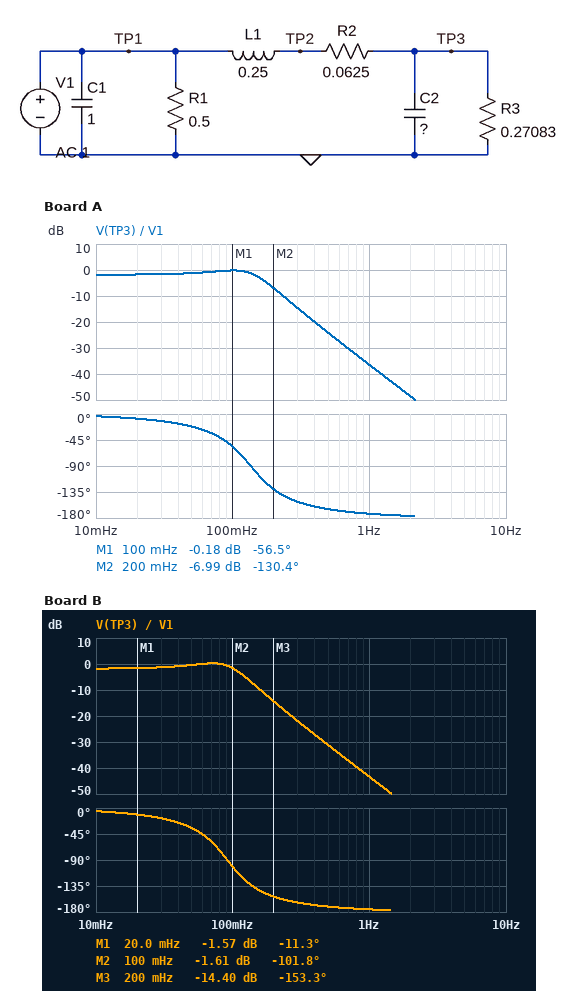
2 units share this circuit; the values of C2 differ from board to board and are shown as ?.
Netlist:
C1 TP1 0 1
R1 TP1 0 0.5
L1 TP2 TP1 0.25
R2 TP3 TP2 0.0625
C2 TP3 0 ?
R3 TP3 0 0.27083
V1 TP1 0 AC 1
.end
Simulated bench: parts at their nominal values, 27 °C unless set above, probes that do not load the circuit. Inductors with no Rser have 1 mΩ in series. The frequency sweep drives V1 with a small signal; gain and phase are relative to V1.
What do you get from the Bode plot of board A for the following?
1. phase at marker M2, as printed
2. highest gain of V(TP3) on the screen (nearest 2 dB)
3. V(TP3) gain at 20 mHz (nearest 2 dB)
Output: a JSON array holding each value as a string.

["-130.4 deg", "0 dB", "-2 dB"]
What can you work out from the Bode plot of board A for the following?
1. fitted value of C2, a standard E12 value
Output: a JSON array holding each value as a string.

["6.8 F"]
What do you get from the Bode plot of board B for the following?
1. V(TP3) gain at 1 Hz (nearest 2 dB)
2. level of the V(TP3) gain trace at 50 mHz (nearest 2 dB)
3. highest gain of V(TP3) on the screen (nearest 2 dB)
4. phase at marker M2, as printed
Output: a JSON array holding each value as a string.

["-44 dB", "0 dB", "0 dB", "-101.8 deg"]
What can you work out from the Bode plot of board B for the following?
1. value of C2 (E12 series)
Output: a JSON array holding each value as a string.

["15 F"]
